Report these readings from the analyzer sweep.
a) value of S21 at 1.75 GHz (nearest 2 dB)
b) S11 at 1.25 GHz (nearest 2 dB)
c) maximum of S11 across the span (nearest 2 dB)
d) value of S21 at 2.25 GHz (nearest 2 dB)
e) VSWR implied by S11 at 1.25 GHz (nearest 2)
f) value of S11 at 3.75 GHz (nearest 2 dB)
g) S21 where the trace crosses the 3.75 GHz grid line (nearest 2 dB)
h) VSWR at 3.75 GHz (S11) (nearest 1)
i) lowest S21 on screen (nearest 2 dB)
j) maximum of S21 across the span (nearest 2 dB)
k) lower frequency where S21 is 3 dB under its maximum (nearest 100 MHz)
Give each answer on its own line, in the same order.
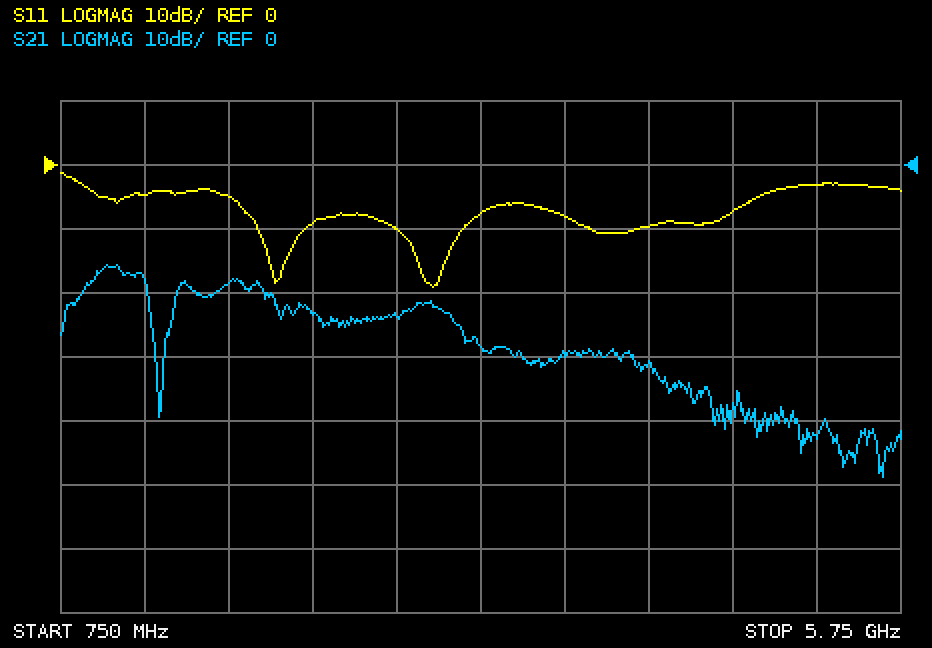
-18 dB
-4 dB
-2 dB
-24 dB
4
-8 dB
-30 dB
2
-48 dB
-16 dB
900 MHz
